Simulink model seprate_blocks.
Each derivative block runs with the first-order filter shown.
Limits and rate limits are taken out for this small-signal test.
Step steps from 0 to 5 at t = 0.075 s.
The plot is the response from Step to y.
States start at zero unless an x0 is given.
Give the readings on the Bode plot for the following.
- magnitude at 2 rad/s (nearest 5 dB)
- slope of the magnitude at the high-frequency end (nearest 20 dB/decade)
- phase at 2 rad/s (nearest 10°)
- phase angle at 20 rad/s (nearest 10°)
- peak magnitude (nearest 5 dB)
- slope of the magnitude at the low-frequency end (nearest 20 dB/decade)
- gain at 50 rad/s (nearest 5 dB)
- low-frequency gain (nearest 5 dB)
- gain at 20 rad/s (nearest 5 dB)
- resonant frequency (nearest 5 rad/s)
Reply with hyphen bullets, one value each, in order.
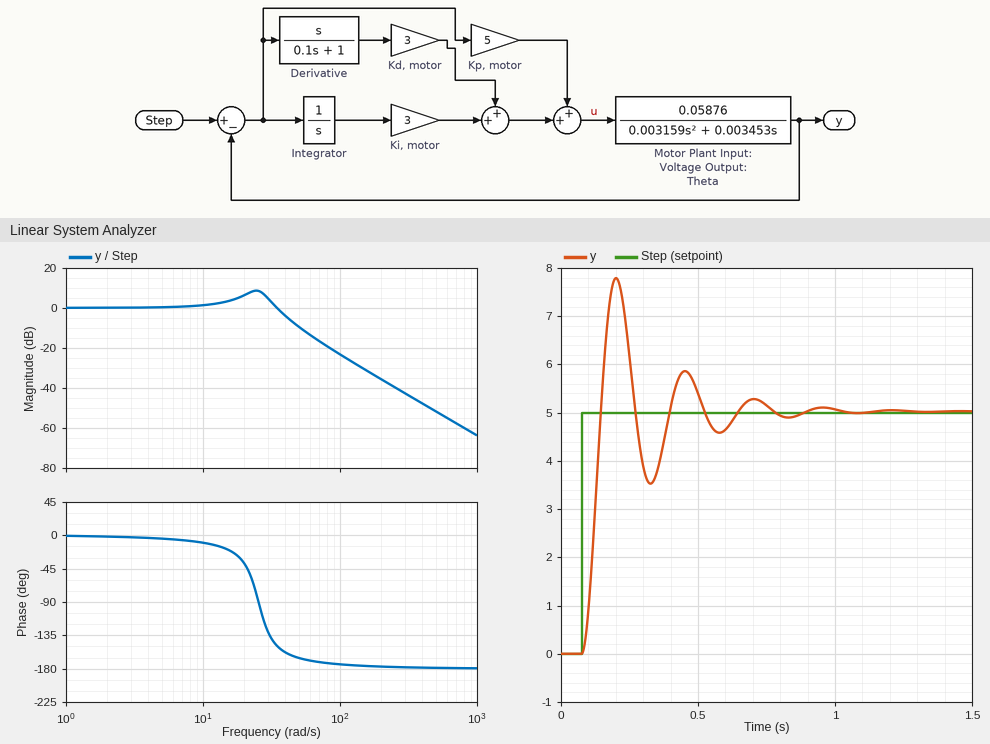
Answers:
- 0 dB
- -40 dB/decade
- 0°
- -40°
- 10 dB
- 0 dB/decade
- -10 dB
- 0 dB
- 5 dB
- 25 rad/s
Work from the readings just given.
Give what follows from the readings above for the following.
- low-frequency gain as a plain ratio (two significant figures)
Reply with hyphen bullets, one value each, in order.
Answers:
- 1.0
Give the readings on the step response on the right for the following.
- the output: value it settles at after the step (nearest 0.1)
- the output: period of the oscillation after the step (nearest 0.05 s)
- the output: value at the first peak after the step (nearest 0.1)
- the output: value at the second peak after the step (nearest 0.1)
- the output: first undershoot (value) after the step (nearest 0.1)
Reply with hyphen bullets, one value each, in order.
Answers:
- 5.0
- 0.25 s
- 7.8
- 5.9
- 3.5
